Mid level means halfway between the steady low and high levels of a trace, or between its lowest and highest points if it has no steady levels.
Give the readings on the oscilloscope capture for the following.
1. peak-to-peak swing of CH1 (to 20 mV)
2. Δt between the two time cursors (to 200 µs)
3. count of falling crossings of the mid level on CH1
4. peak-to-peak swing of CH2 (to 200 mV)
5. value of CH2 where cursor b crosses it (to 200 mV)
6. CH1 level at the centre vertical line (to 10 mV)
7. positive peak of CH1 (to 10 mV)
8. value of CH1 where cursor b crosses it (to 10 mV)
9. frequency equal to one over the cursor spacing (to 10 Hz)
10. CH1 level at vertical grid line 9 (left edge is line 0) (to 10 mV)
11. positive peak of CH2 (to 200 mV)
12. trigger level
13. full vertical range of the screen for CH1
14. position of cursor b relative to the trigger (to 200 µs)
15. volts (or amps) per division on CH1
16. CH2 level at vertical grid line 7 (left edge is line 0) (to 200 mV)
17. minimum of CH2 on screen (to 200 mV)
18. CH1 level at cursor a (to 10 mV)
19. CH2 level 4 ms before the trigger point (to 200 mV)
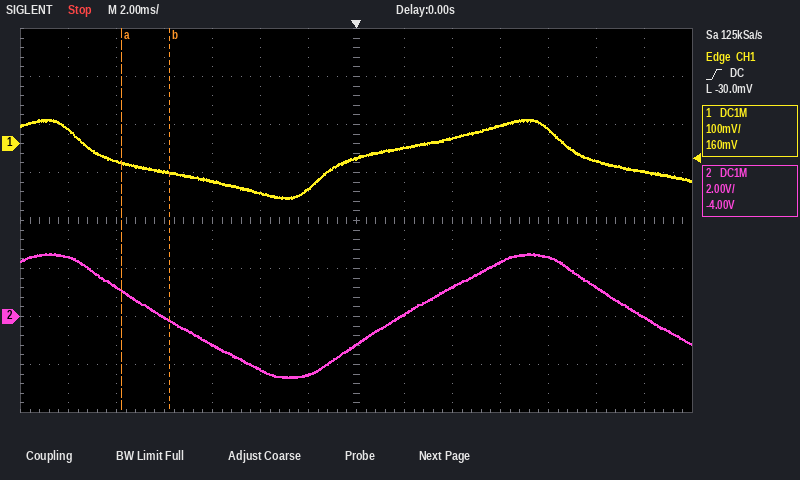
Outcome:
160 mV
2.0 ms
2
5.2 V
-200 mV
-30 mV
50 mV
-60 mV
500 Hz
10 mV
2.6 V
-30.0 mV
800 mV
-7.8 ms
100 mV
-1.2 V
-2.6 V
-40 mV
-2.2 V
